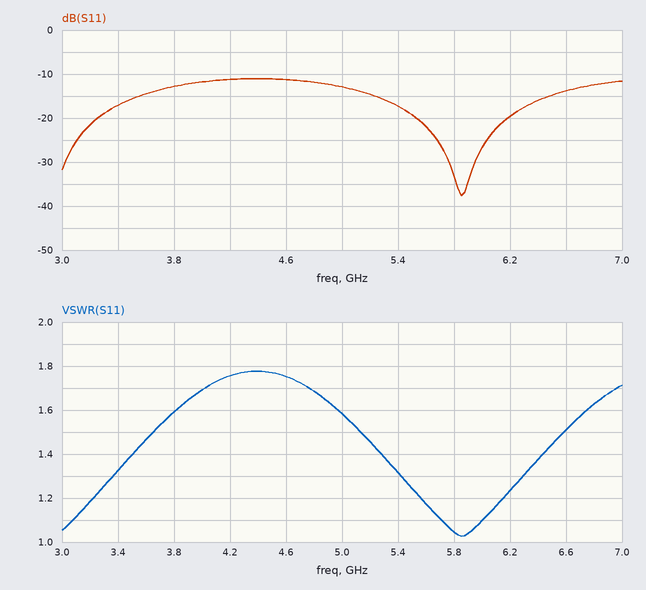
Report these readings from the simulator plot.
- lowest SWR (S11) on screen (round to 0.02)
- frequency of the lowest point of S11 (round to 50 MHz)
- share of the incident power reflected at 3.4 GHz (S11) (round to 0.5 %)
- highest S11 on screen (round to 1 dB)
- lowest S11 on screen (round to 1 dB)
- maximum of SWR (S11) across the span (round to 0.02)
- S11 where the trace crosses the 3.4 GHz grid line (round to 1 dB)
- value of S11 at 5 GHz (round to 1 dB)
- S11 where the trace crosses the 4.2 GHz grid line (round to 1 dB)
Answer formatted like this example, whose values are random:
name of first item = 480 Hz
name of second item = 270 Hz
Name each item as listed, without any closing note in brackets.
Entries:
lowest SWR (S11) on screen = 1.02
frequency of the lowest point of S11 = 5.85 GHz
share of the incident power reflected at 3.4 GHz (S11) = 2.0 %
highest S11 on screen = -11 dB
lowest S11 on screen = -38 dB
maximum of SWR (S11) across the span = 1.78
S11 where the trace crosses the 3.4 GHz grid line = -17 dB
value of S11 at 5 GHz = -13 dB
S11 where the trace crosses the 4.2 GHz grid line = -11 dB
